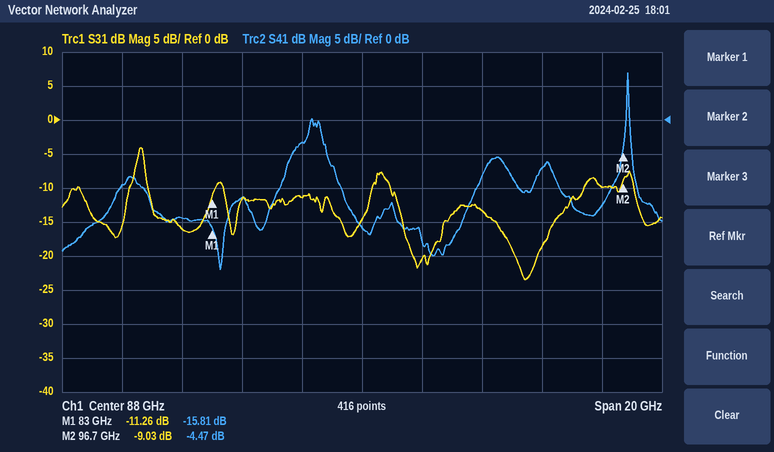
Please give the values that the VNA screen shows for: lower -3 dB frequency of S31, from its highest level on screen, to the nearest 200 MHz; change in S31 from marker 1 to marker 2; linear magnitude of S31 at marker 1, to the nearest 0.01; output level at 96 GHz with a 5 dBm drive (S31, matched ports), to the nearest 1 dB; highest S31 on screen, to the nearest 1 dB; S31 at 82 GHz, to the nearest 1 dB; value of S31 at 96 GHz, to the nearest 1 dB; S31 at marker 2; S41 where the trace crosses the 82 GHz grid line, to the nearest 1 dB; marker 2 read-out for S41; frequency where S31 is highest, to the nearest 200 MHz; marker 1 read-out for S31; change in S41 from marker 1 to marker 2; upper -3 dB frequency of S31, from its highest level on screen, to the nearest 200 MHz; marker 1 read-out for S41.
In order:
80.4 GHz
2.23 dB
0.27
-5 dBm
-4 dB
-16 dB
-10 dB
-9.03 dB
-14 dB
-4.47 dB
80.6 GHz
-11.26 dB
11.34 dB
80.8 GHz
-15.81 dB
